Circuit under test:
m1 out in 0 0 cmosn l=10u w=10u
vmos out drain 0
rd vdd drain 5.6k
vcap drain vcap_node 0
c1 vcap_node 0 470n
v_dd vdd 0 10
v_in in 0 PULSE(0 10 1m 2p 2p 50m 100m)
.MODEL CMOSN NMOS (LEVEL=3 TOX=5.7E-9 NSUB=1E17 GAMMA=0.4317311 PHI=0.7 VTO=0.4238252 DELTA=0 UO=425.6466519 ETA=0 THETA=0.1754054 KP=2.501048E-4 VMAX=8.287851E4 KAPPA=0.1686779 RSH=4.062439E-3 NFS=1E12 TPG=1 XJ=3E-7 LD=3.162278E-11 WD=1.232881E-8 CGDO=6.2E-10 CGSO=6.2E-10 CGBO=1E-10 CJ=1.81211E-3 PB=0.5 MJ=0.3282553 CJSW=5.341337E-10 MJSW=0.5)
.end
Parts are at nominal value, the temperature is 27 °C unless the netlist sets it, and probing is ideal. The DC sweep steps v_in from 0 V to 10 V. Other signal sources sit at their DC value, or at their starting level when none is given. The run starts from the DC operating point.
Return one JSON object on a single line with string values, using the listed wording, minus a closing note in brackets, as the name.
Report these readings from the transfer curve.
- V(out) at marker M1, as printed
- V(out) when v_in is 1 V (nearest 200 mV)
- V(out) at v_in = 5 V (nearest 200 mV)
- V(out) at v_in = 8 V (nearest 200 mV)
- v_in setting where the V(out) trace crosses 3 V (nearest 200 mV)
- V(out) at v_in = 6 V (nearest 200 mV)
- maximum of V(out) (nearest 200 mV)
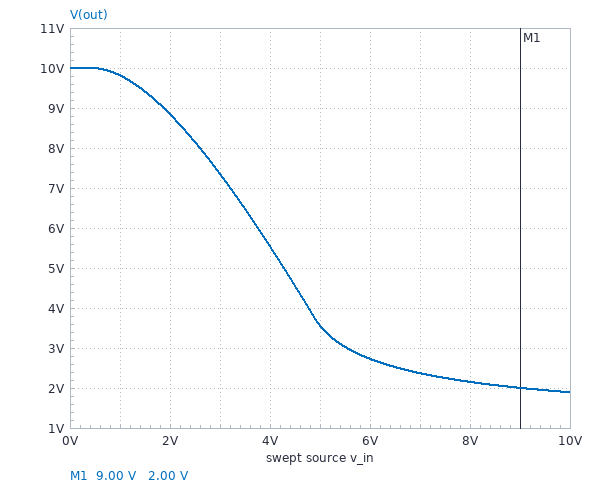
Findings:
{"V(out) at marker M1, as printed": "2.00 V", "V(out) when v_in is 1 V": "9.8 V", "V(out) at v_in = 5 V": "3.6 V", "V(out) at v_in = 8 V": "2.2 V", "v_in setting where the V(out) trace crosses 3 V": "5.6 V", "V(out) at v_in = 6 V": "2.8 V", "maximum of V(out)": "10.0 V"}
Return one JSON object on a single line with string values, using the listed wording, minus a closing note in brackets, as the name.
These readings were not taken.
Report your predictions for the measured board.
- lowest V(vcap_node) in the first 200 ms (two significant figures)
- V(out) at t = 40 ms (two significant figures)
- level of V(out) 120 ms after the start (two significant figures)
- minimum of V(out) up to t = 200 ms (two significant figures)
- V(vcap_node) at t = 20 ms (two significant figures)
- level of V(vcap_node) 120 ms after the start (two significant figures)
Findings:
{"lowest V(vcap_node) in the first 200 ms": "1.9 V", "V(out) at t = 40 ms": "1.9 V", "level of V(out) 120 ms after the start": "1.9 V", "minimum of V(out) up to t = 200 ms": "1.9 V", "V(vcap_node) at t = 20 ms": "1.9 V", "level of V(vcap_node) 120 ms after the start": "1.9 V"}
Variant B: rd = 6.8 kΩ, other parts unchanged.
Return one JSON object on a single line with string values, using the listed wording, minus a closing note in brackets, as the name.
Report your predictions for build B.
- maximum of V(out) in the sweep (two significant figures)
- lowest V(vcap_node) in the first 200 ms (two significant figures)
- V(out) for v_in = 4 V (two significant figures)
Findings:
{"maximum of V(out) in the sweep": "10 V", "lowest V(vcap_node) in the first 200 ms": "1.6 V", "V(out) for v_in = 4 V": "4.6 V"}
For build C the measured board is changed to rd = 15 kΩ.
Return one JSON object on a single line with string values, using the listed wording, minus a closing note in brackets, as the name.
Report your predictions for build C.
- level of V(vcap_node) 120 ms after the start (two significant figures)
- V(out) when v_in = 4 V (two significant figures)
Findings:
{"level of V(vcap_node) 120 ms after the start": "730 mV", "V(out) when v_in = 4 V": "1.4 V"}
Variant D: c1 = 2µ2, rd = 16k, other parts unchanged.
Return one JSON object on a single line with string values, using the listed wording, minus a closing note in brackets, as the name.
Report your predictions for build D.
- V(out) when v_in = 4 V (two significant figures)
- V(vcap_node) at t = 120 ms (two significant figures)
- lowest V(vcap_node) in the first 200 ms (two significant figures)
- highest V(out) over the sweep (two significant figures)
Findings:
{"V(out) when v_in = 4 V": "1.3 V", "V(vcap_node) at t = 120 ms": "700 mV", "lowest V(vcap_node) in the first 200 ms": "690 mV", "highest V(out) over the sweep": "10 V"}
